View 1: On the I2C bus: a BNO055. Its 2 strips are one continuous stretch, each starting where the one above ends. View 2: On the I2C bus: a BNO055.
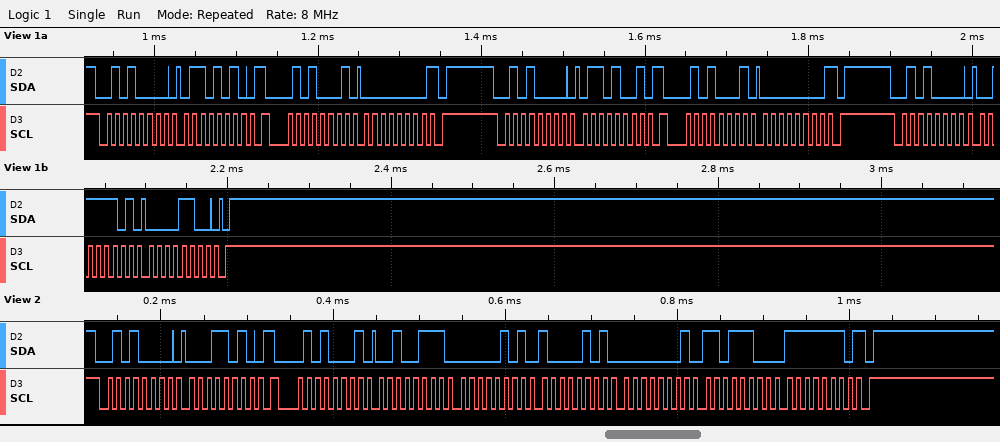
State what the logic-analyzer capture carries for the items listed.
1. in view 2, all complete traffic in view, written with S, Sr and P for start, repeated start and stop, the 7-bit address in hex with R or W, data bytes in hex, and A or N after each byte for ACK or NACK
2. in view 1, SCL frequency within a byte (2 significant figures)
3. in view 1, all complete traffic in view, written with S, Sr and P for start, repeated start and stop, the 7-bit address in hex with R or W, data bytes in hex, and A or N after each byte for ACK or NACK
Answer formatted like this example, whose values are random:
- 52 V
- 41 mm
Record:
- S 28W A 1A A Sr 28R A 27 A 05 A 85 A 01 A DC A FE N P
- 100 kHz
- S 28W A 6A A Sr 28R A 00 N P S 28W A 69 A Sr 28R A 00 N P S 28W A 3D A 0C A P
